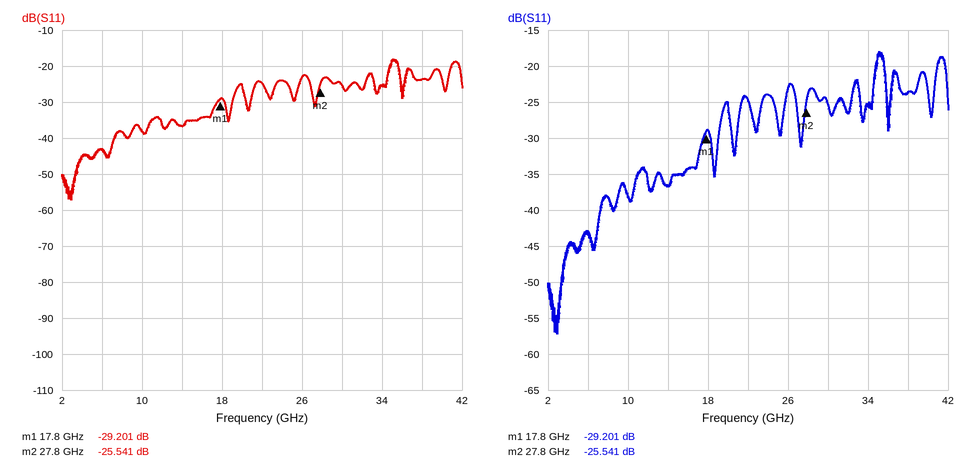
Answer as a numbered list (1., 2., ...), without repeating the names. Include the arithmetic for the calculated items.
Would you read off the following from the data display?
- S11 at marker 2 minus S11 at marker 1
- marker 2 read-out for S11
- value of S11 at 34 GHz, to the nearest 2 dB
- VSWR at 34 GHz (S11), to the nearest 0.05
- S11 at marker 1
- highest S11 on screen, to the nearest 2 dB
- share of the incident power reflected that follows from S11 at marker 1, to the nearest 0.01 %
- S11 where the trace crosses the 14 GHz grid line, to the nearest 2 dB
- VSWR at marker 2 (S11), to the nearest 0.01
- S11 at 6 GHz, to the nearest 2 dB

1. -25.541 − (-29.201) = 3.660 dB
2. -25.541 dB
3. -26 dB
4. |Γ| = 10^(-26/20) = 0.0501; VSWR = (1 + 0.0501)/(1 − 0.0501) ≈ 1.11, so 1.10 to the nearest 0.05
5. -29.201 dB
6. -18 dB
7. 10^(-29.201/10) ≈ 0.12 %
8. -36 dB
9. (1 + 0.0528)/(1 − 0.0528) ≈ 1.11
10. -44 dB
